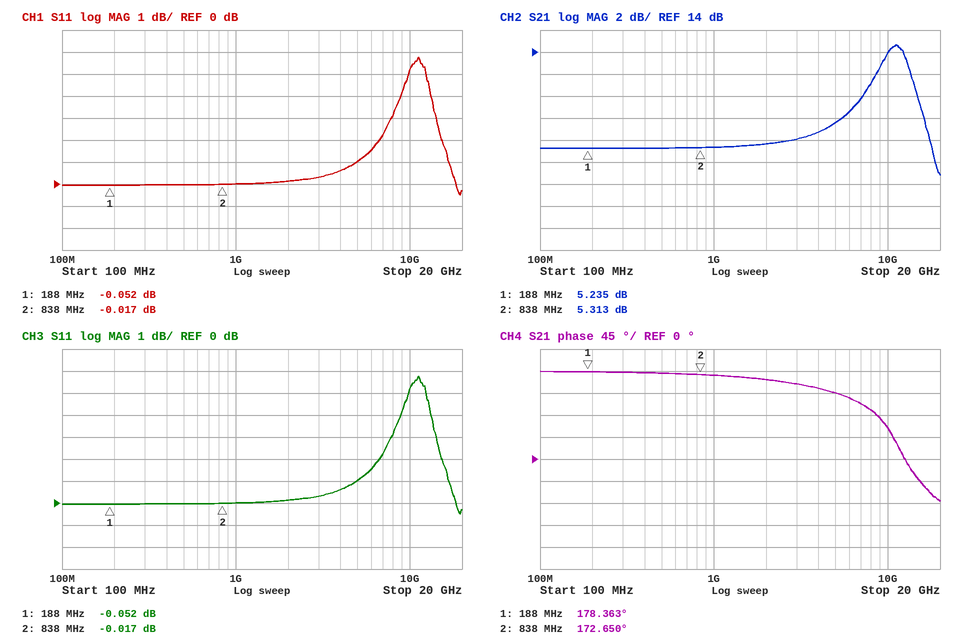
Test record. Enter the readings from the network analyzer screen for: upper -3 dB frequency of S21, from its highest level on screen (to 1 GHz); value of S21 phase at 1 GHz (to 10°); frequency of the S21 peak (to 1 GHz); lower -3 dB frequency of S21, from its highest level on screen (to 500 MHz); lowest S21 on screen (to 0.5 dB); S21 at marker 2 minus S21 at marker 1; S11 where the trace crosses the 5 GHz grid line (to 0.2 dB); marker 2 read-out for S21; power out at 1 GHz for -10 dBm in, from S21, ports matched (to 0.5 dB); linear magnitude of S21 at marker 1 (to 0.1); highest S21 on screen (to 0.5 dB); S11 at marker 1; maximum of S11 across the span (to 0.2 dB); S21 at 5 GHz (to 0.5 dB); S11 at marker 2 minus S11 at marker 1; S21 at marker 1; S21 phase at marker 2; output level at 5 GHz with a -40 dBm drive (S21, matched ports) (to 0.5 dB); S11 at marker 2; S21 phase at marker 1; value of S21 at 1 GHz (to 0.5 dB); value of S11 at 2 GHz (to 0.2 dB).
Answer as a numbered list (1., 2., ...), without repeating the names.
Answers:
1. 14 GHz
2. 170°
3. 11 GHz
4. 8.5 GHz
5. 3.0 dB
6. 0.078 dB
7. 1.0 dB
8. 5.313 dB
9. -4.5 dBm
10. 1.8
11. 14.5 dB
12. -0.052 dB
13. 5.8 dB
14. 7.5 dB
15. 0.035 dB
16. 5.235 dB
17. 172.650°
18. -32.5 dBm
19. -0.017 dB
20. 178.363°
21. 5.5 dB
22. 0.2 dB
